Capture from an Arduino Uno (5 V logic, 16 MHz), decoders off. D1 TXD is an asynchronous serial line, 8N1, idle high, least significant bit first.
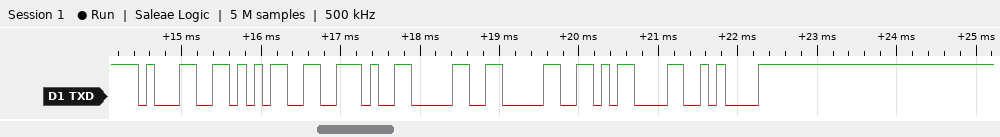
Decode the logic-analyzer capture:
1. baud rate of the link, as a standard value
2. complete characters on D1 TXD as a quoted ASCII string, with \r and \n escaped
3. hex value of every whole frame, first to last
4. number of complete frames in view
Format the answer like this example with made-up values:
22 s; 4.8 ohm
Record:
9600 baud; "15.00\r\n"; 0x31 0x35 0x2E 0x30 0x30 0x0D 0x0A; 7
